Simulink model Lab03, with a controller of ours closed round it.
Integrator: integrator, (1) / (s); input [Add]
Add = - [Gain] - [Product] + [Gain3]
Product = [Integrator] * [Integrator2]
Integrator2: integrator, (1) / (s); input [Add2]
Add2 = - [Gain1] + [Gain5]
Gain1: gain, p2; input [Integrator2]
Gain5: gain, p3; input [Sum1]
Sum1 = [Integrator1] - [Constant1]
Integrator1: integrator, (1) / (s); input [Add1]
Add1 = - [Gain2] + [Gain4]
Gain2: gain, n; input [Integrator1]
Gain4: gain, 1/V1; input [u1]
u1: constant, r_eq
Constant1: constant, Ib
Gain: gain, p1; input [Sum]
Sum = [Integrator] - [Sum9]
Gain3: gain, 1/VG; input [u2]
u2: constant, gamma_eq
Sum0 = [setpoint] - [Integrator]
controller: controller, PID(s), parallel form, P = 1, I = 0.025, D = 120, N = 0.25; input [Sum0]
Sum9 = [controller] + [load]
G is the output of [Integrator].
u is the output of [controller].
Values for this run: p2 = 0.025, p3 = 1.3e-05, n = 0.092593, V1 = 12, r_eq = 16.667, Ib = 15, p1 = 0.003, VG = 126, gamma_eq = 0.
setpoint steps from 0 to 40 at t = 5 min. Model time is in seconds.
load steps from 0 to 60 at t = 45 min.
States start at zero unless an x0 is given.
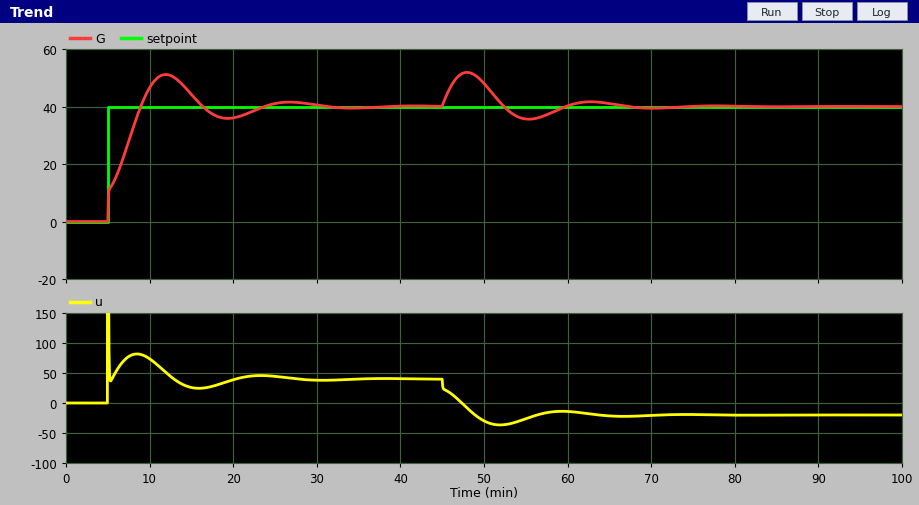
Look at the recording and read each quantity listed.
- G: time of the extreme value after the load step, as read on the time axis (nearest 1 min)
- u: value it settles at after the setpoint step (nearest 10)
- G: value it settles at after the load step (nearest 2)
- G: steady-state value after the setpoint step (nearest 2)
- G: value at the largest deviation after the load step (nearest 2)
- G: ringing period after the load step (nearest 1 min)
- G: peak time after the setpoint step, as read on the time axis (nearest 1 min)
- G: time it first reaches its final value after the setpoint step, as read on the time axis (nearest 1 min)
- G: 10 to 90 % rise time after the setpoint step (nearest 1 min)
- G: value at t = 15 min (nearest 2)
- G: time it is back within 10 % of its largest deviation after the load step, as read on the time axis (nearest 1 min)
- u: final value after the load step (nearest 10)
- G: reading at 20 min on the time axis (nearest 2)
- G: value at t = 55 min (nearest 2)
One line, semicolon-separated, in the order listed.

48 min; 40; 40; 40; 52; 15 min; 12 min; 9 min; 3 min; 44; 65 min; -20; 36; 36
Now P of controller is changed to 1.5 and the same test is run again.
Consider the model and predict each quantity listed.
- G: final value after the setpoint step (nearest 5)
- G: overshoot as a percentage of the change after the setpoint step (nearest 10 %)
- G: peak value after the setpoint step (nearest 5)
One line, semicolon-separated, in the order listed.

40; 20 %; 50
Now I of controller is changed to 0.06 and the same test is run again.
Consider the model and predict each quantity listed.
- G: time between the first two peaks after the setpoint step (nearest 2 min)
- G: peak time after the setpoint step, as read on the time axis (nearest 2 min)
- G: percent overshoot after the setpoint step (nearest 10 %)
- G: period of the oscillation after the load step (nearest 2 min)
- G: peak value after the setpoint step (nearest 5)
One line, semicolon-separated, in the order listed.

10 min; 10 min; 40 %; 10 min; 55
